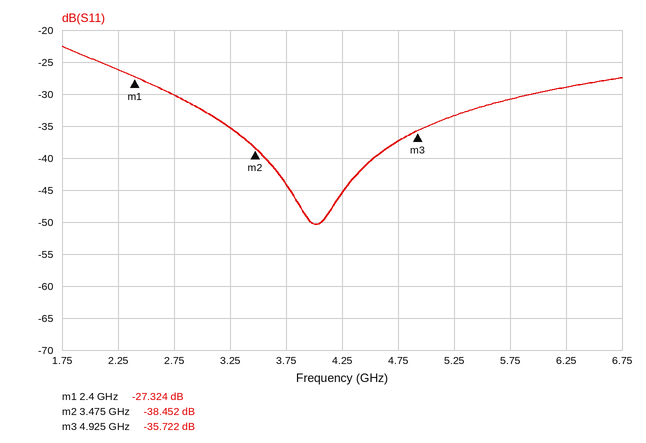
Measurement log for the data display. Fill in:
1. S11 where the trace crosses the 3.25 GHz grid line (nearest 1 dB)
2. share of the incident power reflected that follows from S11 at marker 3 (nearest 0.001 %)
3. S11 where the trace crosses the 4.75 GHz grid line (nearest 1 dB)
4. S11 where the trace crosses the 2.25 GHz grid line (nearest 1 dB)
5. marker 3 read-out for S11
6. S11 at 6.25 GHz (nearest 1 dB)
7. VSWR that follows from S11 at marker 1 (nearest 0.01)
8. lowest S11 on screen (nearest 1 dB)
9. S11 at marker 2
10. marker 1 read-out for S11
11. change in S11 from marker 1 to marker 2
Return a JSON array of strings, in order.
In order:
["-35 dB", "0.027 %", "-37 dB", "-26 dB", "-35.722 dB", "-29 dB", "1.09", "-50 dB", "-38.452 dB", "-27.324 dB", "-11.128 dB"]
